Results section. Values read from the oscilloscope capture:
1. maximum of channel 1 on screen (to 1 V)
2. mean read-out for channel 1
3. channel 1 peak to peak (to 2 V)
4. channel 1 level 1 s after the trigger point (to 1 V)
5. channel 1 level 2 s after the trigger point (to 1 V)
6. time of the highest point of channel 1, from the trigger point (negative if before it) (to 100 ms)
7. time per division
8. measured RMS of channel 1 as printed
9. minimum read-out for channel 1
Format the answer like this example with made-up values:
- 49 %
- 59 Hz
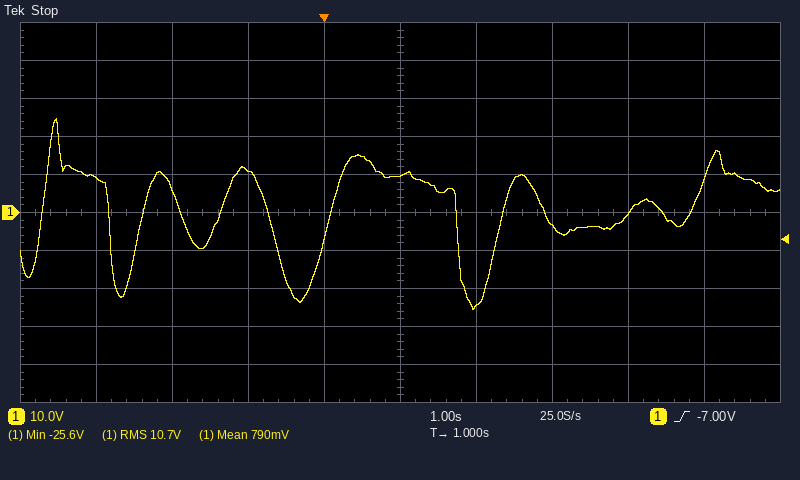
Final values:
- 25 V
- 790 mV
- 50 V
- 10 V
- -25 V
- -3.5 s
- 1 s
- 10.7 V
- -25.6 V
